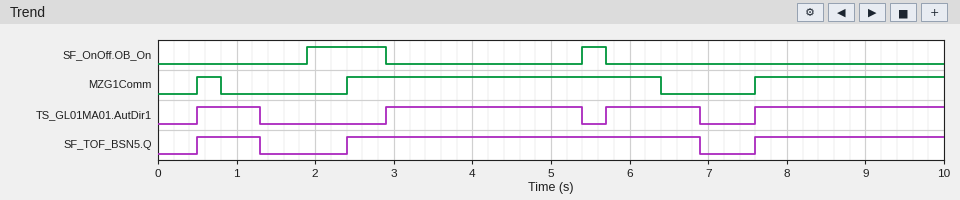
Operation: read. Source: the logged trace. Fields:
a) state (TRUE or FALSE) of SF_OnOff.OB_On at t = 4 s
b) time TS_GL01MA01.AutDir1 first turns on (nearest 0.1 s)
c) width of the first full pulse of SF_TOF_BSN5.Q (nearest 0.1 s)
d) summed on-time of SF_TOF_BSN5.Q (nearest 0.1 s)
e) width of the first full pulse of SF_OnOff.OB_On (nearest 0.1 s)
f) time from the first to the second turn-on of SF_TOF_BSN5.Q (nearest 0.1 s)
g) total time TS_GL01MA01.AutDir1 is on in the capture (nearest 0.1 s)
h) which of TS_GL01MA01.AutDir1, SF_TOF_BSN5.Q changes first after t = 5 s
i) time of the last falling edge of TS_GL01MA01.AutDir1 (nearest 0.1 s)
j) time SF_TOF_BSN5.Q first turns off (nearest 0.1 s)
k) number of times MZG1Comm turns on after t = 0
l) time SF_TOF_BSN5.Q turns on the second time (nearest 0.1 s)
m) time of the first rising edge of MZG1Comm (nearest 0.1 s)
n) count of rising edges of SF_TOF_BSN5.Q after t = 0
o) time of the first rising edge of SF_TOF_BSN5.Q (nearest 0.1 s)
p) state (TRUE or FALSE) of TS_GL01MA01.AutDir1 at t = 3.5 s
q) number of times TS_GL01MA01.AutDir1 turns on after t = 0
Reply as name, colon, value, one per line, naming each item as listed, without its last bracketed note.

state (TRUE or FALSE) of SF_OnOff.OB_On at t = 4 s: FALSE
time TS_GL01MA01.AutDir1 first turns on: 0.5 s
width of the first full pulse of SF_TOF_BSN5.Q: 0.8 s
summed on-time of SF_TOF_BSN5.Q: 7.7 s
width of the first full pulse of SF_OnOff.OB_On: 1.0 s
time from the first to the second turn-on of SF_TOF_BSN5.Q: 1.9 s
total time TS_GL01MA01.AutDir1 is on in the capture: 6.9 s
which of TS_GL01MA01.AutDir1, SF_TOF_BSN5.Q changes first after t = 5 s: TS_GL01MA01.AutDir1
time of the last falling edge of TS_GL01MA01.AutDir1: 6.9 s
time SF_TOF_BSN5.Q first turns off: 1.3 s
number of times MZG1Comm turns on after t = 0: 3
time SF_TOF_BSN5.Q turns on the second time: 2.4 s
time of the first rising edge of MZG1Comm: 0.5 s
count of rising edges of SF_TOF_BSN5.Q after t = 0: 3
time of the first rising edge of SF_TOF_BSN5.Q: 0.5 s
state (TRUE or FALSE) of TS_GL01MA01.AutDir1 at t = 3.5 s: TRUE
number of times TS_GL01MA01.AutDir1 turns on after t = 0: 4
